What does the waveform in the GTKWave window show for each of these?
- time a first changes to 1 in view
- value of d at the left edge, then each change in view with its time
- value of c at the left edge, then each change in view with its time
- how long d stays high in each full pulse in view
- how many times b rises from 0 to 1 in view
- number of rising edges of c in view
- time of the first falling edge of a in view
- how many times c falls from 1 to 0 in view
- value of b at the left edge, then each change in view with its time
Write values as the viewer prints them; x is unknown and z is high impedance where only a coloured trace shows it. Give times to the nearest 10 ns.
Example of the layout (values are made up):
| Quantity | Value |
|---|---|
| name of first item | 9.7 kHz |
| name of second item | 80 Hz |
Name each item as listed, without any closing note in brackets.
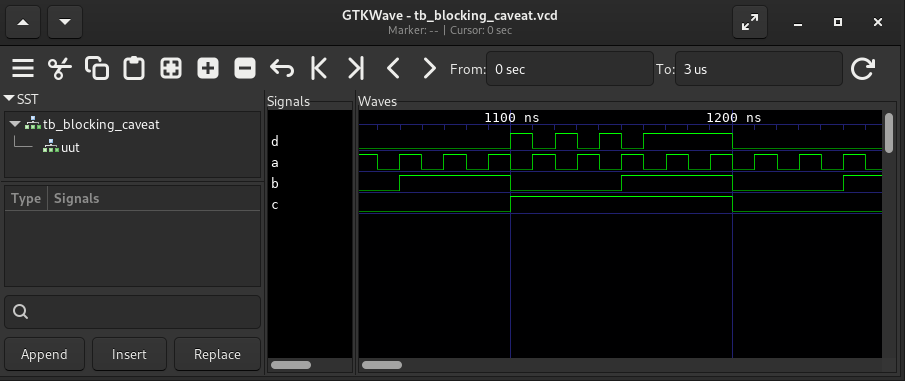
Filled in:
| Quantity | Value |
|---|---|
| time a first changes to 1 in view | 1050 ns |
| value of d at the left edge, then each change in view with its time | 0, 1 at 1100 ns, 0 at 1110 ns, 1 at 1120 ns, 0 at 1130 ns, 1 at 1140 ns, 0 at 1150 ns, 1 at 1160 ns, 0 at 1200 ns |
| value of c at the left edge, then each change in view with its time | 0, 1 at 1100 ns, 0 at 1200 ns |
| how long d stays high in each full pulse in view | 10 ns, 10 ns, 10 ns, 40 ns |
| how many times b rises from 0 to 1 in view | 3 |
| number of rising edges of c in view | 1 |
| time of the first falling edge of a in view | 1040 ns |
| how many times c falls from 1 to 0 in view | 1 |
| value of b at the left edge, then each change in view with its time | 0, 1 at 1050 ns, 0 at 1100 ns, 1 at 1150 ns, 0 at 1200 ns, 1 at 1250 ns |
